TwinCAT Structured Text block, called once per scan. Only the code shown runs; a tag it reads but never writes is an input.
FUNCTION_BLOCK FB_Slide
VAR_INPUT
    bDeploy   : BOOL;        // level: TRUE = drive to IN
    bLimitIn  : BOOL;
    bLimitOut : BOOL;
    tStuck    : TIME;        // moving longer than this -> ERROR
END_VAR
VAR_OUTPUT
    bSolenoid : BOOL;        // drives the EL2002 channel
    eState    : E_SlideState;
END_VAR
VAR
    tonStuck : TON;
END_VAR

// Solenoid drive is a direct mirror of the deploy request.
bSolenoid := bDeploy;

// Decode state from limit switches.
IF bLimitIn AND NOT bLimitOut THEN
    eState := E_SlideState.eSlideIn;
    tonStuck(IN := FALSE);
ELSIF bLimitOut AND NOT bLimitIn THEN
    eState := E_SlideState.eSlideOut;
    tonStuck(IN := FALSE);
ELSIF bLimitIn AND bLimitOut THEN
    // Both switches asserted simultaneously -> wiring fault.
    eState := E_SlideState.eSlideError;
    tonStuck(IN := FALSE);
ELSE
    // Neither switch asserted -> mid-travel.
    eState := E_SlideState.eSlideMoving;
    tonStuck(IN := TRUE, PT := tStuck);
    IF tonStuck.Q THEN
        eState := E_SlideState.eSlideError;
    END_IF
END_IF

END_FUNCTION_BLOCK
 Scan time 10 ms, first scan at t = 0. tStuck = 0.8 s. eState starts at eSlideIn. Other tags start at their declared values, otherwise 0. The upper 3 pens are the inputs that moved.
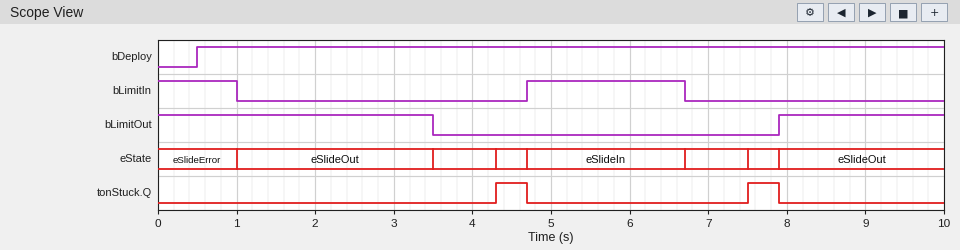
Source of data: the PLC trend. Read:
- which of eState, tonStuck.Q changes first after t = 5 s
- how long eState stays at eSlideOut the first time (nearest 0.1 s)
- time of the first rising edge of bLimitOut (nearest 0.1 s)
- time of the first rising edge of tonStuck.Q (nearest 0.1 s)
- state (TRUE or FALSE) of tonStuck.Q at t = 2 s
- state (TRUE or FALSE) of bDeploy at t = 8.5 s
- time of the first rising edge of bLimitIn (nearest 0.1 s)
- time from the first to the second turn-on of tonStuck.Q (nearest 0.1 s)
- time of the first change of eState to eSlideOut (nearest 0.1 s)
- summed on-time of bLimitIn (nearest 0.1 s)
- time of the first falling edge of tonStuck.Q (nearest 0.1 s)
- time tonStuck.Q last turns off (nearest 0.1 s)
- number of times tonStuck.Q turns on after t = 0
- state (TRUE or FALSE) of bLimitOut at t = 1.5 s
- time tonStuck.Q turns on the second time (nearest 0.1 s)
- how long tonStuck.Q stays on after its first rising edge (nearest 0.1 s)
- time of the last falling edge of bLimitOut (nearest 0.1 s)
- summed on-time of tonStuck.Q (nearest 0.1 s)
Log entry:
eState
2.5 s
7.9 s
4.3 s
FALSE
TRUE
4.7 s
3.2 s
1.0 s
3.0 s
4.7 s
7.9 s
2
TRUE
7.5 s
0.4 s
3.5 s
0.8 s
